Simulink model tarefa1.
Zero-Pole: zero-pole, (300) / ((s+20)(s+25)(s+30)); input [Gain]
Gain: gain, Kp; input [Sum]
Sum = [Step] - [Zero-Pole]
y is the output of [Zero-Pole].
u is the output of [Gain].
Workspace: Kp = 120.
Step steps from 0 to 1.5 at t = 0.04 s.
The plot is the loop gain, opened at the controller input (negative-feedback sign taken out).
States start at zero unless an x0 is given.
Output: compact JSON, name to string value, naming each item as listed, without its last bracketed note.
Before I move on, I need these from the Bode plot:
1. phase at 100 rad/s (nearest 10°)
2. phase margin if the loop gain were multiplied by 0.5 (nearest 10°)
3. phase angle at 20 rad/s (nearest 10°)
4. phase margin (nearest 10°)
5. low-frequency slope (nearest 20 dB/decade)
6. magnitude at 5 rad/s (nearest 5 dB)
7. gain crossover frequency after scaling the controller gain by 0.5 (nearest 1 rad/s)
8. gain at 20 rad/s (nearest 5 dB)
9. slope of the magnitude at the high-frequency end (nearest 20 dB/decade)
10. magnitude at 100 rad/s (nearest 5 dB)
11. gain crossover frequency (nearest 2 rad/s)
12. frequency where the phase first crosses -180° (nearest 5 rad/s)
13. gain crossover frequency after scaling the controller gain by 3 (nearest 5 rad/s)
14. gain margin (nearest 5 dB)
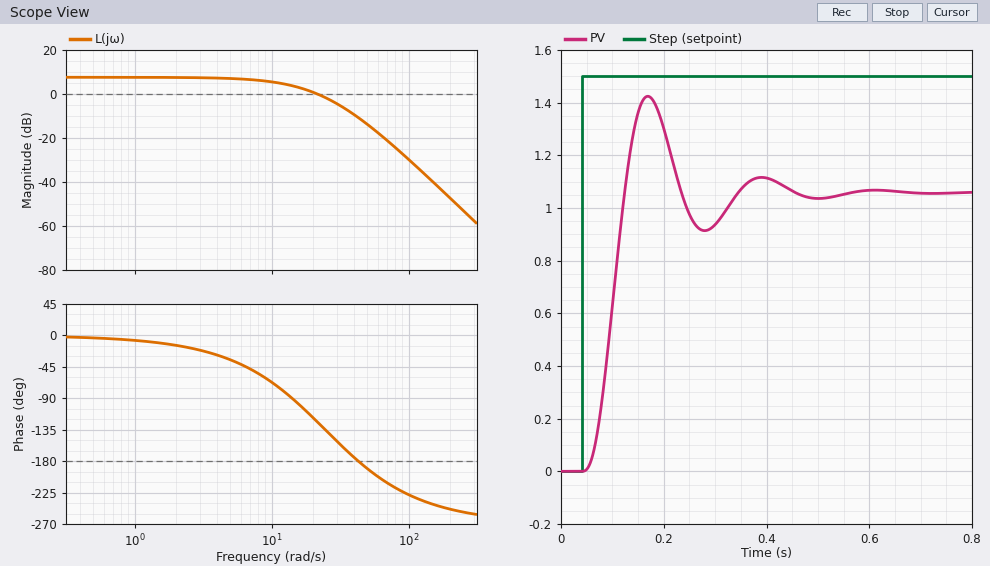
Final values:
{"phase at 100 rad/s": "-230°", "phase margin if the loop gain were multiplied by 0.5": "120°", "phase angle at 20 rad/s": "-120°", "phase margin": "60°", "low-frequency slope": "0 dB/decade", "magnitude at 5 rad/s": "5 dB", "gain crossover frequency after scaling the controller gain by 0.5": "9 rad/s", "gain at 20 rad/s": "0 dB", "slope of the magnitude at the high-frequency end": "-60 dB/decade", "magnitude at 100 rad/s": "-30 dB", "gain crossover frequency": "22 rad/s", "frequency where the phase first crosses -180°": "45 rad/s", "gain crossover frequency after scaling the controller gain by 3": "40 rad/s", "gain margin": "10 dB"}
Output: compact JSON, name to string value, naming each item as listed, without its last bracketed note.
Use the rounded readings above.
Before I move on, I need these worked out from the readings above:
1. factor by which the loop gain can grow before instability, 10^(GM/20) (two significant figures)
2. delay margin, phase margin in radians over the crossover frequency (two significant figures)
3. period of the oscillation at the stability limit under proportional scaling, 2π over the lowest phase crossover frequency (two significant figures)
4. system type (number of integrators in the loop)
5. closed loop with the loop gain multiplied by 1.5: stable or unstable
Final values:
{"factor by which the loop gain can grow before instability, 10^(GM/20)": "3.2", "delay margin, phase margin in radians over the crossover frequency": "0.048 s", "period of the oscillation at the stability limit under proportional scaling, 2π over the lowest phase crossover frequency": "0.14 s", "system type": "0", "closed loop with the loop gain multiplied by 1.5: stable or unstable": "stable"}
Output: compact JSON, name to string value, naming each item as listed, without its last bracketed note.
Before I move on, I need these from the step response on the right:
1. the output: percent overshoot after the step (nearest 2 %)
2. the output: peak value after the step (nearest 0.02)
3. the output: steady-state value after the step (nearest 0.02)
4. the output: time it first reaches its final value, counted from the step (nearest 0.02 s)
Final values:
{"the output: percent overshoot after the step": "34 %", "the output: peak value after the step": "1.42", "the output: steady-state value after the step": "1.06", "the output: time it first reaches its final value, counted from the step": "0.08 s"}
